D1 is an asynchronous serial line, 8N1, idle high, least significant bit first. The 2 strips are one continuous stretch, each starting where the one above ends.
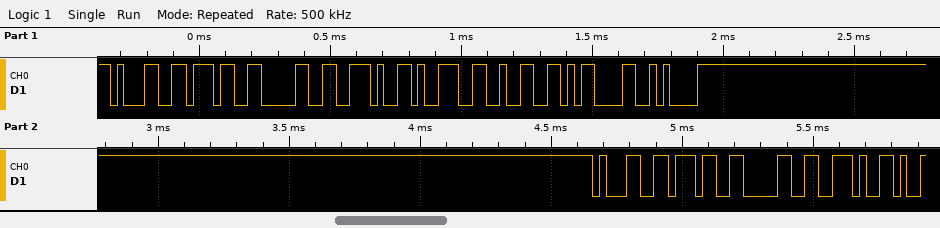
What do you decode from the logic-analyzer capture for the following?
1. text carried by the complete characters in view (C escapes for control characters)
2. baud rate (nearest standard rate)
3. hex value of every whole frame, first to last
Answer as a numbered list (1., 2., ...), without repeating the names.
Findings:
1. "170.92\r\n170."
2. 38400 baud
3. 31 37 30 2E 39 32 0D 0A 31 37 30 2E
